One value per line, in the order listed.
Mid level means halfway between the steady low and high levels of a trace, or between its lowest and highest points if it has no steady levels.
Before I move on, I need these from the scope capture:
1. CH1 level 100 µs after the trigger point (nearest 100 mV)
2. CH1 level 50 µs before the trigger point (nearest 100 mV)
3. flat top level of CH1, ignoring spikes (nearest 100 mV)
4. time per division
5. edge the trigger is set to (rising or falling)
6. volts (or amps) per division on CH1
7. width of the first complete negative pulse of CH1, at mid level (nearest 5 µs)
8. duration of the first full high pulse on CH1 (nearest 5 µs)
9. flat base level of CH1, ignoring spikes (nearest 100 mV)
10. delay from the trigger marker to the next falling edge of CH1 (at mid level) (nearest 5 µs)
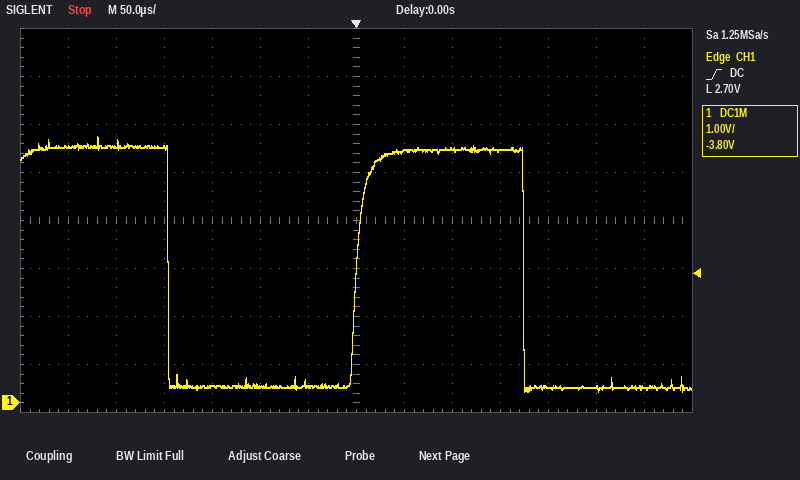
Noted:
5.3 V
300 mV
5.3 V
50 µs
rising
1 V
195 µs
175 µs
300 mV
175 µs
